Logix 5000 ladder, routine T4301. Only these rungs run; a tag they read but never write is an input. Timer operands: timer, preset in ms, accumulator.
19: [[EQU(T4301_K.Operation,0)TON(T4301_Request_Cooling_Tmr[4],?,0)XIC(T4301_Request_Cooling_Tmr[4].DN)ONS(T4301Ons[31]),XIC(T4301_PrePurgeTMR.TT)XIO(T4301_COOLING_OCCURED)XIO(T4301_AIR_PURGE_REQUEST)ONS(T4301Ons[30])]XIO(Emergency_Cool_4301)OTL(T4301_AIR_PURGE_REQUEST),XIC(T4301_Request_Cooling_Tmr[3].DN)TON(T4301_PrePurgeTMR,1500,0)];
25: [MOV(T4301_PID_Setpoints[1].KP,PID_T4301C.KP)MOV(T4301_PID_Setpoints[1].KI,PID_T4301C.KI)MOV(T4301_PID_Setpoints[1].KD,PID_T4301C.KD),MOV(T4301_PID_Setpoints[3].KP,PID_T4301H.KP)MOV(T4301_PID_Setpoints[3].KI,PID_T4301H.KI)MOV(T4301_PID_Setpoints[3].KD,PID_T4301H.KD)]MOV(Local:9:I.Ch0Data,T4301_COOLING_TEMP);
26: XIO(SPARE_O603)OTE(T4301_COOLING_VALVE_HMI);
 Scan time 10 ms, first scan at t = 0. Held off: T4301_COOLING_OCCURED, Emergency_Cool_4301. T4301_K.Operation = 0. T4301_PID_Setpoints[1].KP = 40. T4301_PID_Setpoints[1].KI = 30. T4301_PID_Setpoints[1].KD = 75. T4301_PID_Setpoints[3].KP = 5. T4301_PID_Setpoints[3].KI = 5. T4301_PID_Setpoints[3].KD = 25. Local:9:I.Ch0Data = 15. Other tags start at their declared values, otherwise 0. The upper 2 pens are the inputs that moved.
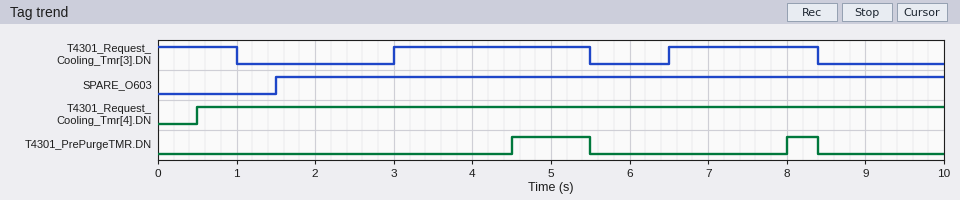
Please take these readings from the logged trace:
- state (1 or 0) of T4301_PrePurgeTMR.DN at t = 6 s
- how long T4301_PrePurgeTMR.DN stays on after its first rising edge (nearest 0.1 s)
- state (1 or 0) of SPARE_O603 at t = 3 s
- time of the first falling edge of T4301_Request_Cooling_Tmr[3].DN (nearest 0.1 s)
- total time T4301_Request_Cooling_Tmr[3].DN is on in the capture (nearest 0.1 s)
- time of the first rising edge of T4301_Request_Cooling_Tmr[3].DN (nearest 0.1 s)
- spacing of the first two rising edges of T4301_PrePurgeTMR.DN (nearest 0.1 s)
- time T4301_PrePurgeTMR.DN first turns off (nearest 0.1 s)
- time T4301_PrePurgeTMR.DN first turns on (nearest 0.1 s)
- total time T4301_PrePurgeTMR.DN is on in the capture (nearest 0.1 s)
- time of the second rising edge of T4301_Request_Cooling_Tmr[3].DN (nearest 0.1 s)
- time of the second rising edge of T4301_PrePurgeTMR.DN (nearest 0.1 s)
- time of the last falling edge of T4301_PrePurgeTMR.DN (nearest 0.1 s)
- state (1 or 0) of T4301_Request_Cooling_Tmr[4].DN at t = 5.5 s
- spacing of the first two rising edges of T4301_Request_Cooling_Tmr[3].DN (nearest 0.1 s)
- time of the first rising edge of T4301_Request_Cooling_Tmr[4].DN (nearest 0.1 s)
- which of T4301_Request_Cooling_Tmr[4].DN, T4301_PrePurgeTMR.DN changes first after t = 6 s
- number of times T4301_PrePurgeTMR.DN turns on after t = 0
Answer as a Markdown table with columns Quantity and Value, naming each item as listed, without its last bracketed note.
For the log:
| Quantity | Value |
|---|---|
| state (1 or 0) of T4301_PrePurgeTMR.DN at t = 6 s | 0 |
| how long T4301_PrePurgeTMR.DN stays on after its first rising edge | 1.0 s |
| state (1 or 0) of SPARE_O603 at t = 3 s | 1 |
| time of the first falling edge of T4301_Request_Cooling_Tmr[3].DN | 1.0 s |
| total time T4301_Request_Cooling_Tmr[3].DN is on in the capture | 5.4 s |
| time of the first rising edge of T4301_Request_Cooling_Tmr[3].DN | 3.0 s |
| spacing of the first two rising edges of T4301_PrePurgeTMR.DN | 3.5 s |
| time T4301_PrePurgeTMR.DN first turns off | 5.5 s |
| time T4301_PrePurgeTMR.DN first turns on | 4.5 s |
| total time T4301_PrePurgeTMR.DN is on in the capture | 1.4 s |
| time of the second rising edge of T4301_Request_Cooling_Tmr[3].DN | 6.5 s |
| time of the second rising edge of T4301_PrePurgeTMR.DN | 8.0 s |
| time of the last falling edge of T4301_PrePurgeTMR.DN | 8.4 s |
| state (1 or 0) of T4301_Request_Cooling_Tmr[4].DN at t = 5.5 s | 1 |
| spacing of the first two rising edges of T4301_Request_Cooling_Tmr[3].DN | 3.5 s |
| time of the first rising edge of T4301_Request_Cooling_Tmr[4].DN | 0.5 s |
| which of T4301_Request_Cooling_Tmr[4].DN, T4301_PrePurgeTMR.DN changes first after t = 6 s | T4301_PrePurgeTMR.DN |
| number of times T4301_PrePurgeTMR.DN turns on after t = 0 | 2 |
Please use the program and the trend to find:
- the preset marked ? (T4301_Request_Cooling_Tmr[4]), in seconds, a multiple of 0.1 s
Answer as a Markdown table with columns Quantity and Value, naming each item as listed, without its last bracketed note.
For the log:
| Quantity | Value |
|---|---|
| the preset marked ? (T4301_Request_Cooling_Tmr[4]), in seconds, a multiple of 0.1 s | 0.5 s |
